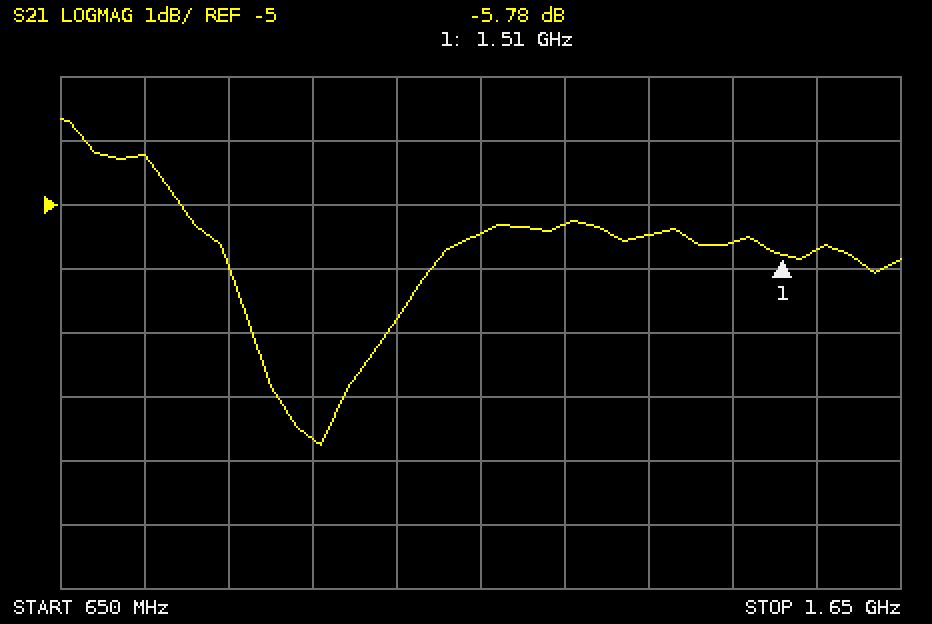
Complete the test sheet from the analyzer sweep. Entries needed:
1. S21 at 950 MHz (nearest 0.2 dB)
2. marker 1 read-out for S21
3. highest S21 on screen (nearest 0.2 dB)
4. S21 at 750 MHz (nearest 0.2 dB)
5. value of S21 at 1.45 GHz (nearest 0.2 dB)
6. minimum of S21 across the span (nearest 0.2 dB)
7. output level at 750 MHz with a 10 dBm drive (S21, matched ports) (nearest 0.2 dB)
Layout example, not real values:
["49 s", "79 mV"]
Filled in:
["-8.6 dB", "-5.78 dB", "-3.6 dB", "-4.2 dB", "-5.6 dB", "-8.8 dB", "5.8 dBm"]
